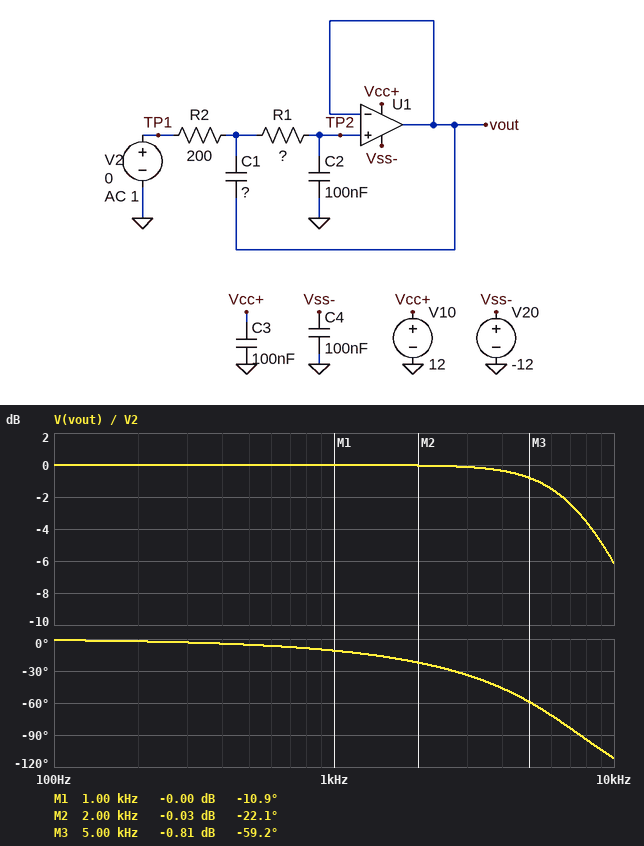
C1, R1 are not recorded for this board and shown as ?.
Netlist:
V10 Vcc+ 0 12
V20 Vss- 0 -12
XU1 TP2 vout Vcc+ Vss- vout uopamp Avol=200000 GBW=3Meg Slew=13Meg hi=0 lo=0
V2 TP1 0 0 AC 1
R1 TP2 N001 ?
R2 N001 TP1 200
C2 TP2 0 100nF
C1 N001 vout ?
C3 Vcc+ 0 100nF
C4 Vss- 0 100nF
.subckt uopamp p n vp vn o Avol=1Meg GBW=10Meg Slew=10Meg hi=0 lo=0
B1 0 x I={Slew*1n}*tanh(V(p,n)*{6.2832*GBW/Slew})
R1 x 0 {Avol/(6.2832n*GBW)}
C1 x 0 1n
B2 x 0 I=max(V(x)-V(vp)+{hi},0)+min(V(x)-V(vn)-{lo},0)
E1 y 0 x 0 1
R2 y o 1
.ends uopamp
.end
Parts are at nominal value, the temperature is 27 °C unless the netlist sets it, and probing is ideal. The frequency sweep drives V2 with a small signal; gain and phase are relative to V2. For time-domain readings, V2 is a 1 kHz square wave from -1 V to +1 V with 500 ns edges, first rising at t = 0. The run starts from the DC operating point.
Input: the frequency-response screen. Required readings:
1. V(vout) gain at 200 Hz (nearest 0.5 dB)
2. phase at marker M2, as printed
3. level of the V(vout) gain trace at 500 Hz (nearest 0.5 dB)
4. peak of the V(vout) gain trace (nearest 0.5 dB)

0 dB
-22.1 deg
0 dB
0 dB
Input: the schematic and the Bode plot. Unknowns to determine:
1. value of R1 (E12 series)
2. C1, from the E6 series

100 Ω
220 nF
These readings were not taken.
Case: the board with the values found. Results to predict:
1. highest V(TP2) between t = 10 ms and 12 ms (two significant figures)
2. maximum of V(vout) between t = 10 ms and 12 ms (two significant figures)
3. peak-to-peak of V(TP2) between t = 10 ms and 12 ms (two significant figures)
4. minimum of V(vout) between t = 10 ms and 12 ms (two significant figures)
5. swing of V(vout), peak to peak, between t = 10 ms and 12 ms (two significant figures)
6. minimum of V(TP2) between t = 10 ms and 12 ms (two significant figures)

1.1 V
1.1 V
2.2 V
-1.1 V
2.2 V
-1.1 V
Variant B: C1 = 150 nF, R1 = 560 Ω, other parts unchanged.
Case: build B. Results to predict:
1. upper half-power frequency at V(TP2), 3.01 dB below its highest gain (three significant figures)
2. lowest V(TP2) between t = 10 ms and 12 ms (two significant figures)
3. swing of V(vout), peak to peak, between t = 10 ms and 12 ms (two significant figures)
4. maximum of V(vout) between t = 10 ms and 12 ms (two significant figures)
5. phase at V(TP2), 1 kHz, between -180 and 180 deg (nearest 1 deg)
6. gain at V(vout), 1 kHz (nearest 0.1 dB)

2.78 kHz
-1.0 V
2.0 V
1.0 V
-27 deg
-0.4 dB
